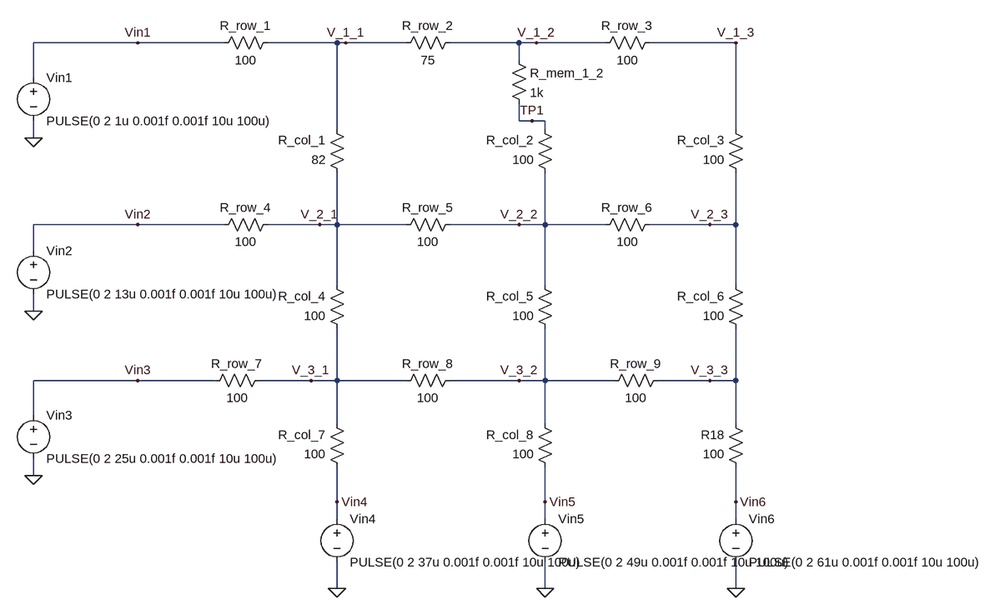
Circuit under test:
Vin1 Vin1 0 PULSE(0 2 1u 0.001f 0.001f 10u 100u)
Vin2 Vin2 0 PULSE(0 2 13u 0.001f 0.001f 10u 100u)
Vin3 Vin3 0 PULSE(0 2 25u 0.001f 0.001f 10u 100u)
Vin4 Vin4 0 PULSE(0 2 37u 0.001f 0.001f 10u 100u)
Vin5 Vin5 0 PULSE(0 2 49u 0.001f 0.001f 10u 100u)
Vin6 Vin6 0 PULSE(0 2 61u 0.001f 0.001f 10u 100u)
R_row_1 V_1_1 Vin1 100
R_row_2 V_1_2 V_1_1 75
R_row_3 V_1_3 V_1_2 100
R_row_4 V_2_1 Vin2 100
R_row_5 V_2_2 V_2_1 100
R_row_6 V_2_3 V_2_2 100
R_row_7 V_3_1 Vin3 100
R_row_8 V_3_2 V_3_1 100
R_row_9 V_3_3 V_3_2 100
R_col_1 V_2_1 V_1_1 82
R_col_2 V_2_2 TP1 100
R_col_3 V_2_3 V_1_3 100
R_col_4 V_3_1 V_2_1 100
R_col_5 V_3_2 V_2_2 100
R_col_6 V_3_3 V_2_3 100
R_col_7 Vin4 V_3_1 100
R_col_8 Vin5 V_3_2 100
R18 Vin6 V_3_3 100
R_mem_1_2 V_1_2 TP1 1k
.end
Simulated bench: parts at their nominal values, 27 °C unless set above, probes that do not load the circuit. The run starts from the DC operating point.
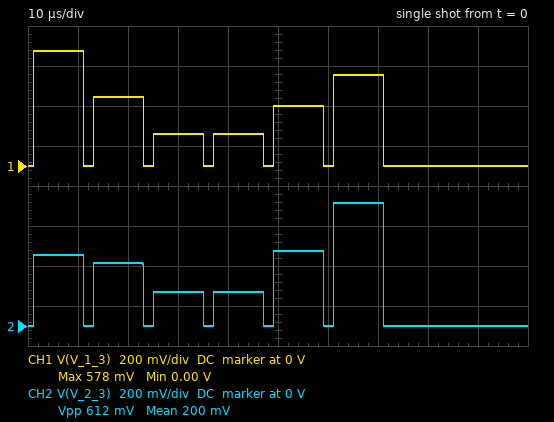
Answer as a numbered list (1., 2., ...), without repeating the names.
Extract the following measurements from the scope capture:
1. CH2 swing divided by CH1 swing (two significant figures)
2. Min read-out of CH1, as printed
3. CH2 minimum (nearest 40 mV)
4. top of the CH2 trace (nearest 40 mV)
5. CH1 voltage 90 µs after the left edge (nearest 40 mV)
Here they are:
1. 1.1
2. 0.00 V
3. 0 V
4. 600 mV
5. 0 V
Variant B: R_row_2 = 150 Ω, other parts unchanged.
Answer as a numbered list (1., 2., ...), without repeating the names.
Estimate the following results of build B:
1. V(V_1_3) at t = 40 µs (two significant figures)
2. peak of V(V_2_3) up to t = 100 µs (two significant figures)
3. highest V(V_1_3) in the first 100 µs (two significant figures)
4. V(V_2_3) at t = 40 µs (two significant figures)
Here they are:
1. 170 mV
2. 630 mV
3. 510 mV
4. 170 mV
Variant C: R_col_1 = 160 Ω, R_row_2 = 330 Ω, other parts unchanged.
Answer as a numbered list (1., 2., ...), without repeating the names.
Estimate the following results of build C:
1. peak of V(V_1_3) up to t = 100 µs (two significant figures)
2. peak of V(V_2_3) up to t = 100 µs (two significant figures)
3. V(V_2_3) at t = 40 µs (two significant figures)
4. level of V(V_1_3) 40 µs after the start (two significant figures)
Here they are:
1. 560 mV
2. 660 mV
3. 180 mV
4. 170 mV
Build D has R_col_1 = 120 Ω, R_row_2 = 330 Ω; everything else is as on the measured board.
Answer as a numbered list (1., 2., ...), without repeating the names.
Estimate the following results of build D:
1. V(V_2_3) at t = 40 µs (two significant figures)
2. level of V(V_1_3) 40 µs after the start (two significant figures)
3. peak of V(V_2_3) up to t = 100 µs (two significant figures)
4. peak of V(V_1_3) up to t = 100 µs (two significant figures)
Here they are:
1. 180 mV
2. 170 mV
3. 660 mV
4. 560 mV
